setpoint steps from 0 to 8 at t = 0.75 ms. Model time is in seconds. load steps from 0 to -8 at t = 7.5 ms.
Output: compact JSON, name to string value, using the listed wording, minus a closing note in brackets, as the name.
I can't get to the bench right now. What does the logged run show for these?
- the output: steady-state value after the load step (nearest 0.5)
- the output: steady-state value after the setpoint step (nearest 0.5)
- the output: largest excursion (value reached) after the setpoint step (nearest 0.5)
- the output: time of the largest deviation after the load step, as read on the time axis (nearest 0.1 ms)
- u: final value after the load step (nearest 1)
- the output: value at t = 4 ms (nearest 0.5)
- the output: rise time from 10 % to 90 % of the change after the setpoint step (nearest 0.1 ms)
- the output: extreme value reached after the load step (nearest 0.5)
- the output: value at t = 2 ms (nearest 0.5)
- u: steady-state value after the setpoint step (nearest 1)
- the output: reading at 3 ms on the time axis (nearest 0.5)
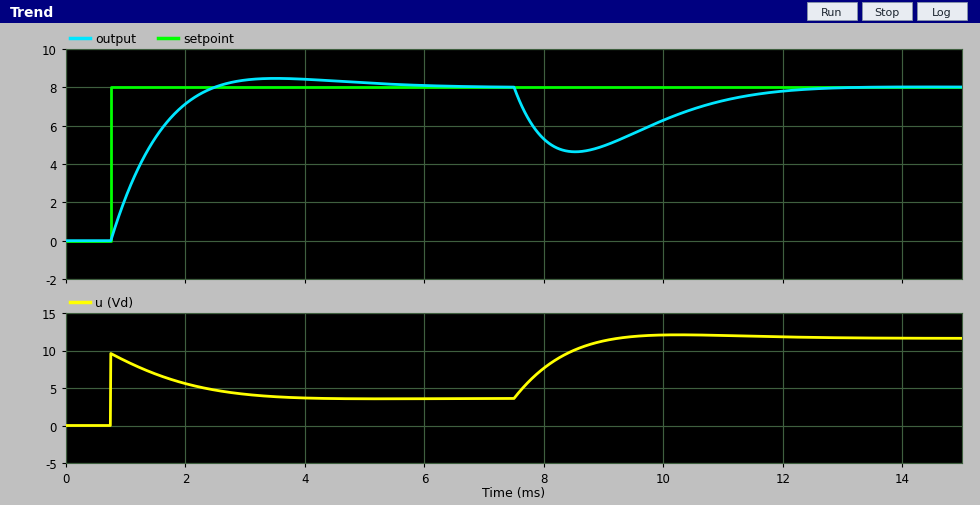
{"the output: steady-state value after the load step": "8.0", "the output: steady-state value after the setpoint step": "8.0", "the output: largest excursion (value reached) after the setpoint step": "8.5", "the output: time of the largest deviation after the load step, as read on the time axis": "8.5 ms", "u: final value after the load step": "12", "the output: value at t = 4 ms": "8.5", "the output: rise time from 10 % to 90 % of the change after the setpoint step": "1.2 ms", "the output: extreme value reached after the load step": "4.5", "the output: value at t = 2 ms": "7.0", "u: steady-state value after the setpoint step": "4", "the output: reading at 3 ms on the time axis": "8.5"}
